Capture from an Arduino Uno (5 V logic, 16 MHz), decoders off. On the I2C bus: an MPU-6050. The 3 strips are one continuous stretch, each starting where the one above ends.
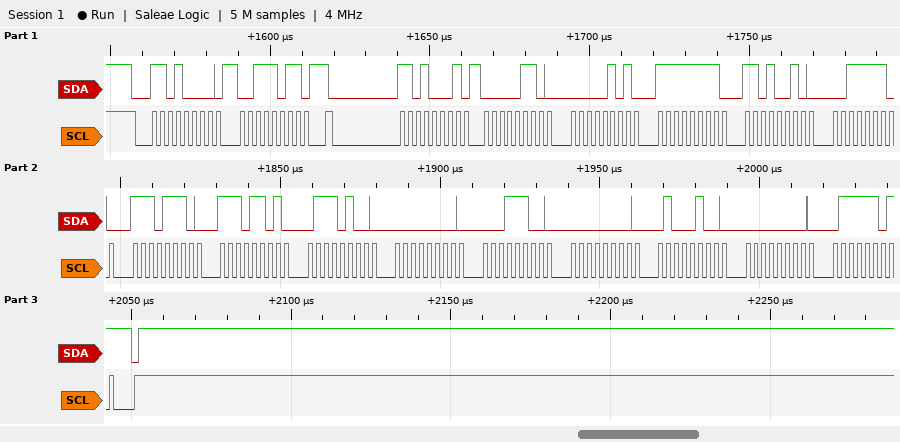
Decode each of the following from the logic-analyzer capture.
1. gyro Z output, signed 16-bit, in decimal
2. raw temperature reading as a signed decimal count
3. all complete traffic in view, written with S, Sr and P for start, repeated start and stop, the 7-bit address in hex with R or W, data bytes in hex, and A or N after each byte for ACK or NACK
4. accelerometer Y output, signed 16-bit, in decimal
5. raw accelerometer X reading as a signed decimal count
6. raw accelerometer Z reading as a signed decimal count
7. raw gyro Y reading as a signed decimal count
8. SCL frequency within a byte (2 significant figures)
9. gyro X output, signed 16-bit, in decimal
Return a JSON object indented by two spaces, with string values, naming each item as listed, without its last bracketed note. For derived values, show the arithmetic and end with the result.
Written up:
{
  "gyro Z output, signed 16-bit, in decimal": "0x007D = 125",
  "raw temperature reading as a signed decimal count": "0xED74 = -4748",
  "all complete traffic in view, written with S, Sr and P for start, repeated start and stop, the 7-bit address in hex with R or W, data bytes in hex, and A or N after each byte for ACK or NACK": "S 68W A 3B A Sr 68R A 06 A 05 A FF A D2 A 3E A EE A ED A 74 A 00 A 1C A 00 A 44 A 00 A 7D N P",
  "accelerometer Y output, signed 16-bit, in decimal": "0xFFD2 = -46",
  "raw accelerometer X reading as a signed decimal count": "0x0605 = 1541",
  "raw accelerometer Z reading as a signed decimal count": "0x3EEE = 16110",
  "raw gyro Y reading as a signed decimal count": "0x0044 = 68",
  "SCL frequency within a byte": "400 kHz",
  "gyro X output, signed 16-bit, in decimal": "0x001C = 28"
}
